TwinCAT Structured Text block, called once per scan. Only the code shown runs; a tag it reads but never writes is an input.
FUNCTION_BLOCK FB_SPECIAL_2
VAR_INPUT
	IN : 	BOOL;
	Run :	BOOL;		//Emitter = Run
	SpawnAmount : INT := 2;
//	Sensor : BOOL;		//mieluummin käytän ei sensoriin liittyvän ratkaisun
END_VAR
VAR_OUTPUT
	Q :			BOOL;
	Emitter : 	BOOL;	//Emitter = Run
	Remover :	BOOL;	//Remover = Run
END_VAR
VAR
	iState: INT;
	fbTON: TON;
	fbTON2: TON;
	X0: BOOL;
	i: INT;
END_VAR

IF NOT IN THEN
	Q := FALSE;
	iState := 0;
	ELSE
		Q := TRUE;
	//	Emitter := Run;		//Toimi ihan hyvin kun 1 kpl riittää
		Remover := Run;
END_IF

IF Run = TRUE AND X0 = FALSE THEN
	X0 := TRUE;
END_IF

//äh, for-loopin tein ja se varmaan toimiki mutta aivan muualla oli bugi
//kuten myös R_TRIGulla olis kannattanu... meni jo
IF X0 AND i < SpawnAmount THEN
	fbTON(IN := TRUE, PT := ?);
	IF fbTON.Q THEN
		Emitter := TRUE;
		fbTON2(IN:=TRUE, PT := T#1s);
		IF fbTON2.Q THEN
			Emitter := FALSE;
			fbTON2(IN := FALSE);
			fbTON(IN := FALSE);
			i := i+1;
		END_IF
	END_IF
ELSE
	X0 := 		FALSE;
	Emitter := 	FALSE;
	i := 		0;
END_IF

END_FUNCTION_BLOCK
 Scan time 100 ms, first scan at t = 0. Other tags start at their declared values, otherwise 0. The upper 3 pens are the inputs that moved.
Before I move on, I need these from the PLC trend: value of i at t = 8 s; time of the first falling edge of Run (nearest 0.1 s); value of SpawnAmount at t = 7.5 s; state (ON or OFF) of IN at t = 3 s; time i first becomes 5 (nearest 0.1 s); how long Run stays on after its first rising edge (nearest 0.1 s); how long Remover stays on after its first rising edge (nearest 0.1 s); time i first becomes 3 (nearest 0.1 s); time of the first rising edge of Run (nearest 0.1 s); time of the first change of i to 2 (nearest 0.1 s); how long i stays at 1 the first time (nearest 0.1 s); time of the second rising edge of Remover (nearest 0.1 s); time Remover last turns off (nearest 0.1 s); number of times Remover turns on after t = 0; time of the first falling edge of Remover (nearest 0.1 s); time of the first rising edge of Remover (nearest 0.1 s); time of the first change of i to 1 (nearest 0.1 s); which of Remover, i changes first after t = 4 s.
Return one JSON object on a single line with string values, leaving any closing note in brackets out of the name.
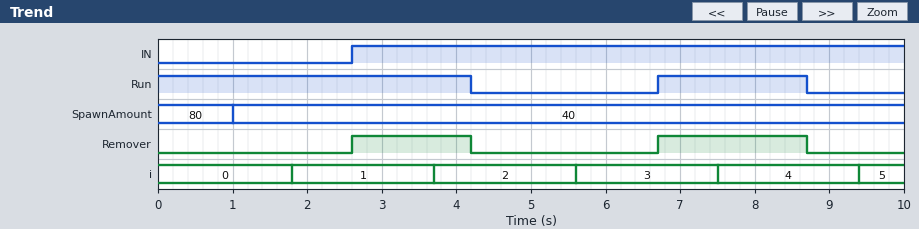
{"value of i at t = 8 s": "4", "time of the first falling edge of Run": "4.2 s", "value of SpawnAmount at t = 7.5 s": "40", "state (ON or OFF) of IN at t = 3 s": "ON", "time i first becomes 5": "9.4 s", "how long Run stays on after its first rising edge": "2.0 s", "how long Remover stays on after its first rising edge": "1.6 s", "time i first becomes 3": "5.6 s", "time of the first rising edge of Run": "6.7 s", "time of the first change of i to 2": "3.7 s", "how long i stays at 1 the first time": "1.9 s", "time of the second rising edge of Remover": "6.7 s", "time Remover last turns off": "8.7 s", "number of times Remover turns on after t = 0": "2", "time of the first falling edge of Remover": "4.2 s", "time of the first rising edge of Remover": "2.6 s", "time of the first change of i to 1": "1.8 s", "which of Remover, i changes first after t = 4 s": "Remover"}
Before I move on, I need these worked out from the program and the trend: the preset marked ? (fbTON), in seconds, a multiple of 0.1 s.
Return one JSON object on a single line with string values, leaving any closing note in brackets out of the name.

{"the preset marked ? (fbTON), in seconds, a multiple of 0.1 s": "0.8 s"}
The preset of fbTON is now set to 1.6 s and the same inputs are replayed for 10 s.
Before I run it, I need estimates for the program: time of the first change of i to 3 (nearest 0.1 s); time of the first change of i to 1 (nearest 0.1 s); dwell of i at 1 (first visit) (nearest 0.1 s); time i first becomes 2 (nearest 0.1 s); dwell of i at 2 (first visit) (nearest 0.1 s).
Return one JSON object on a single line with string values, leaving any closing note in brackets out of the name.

{"time of the first change of i to 3": "8.0 s", "time of the first change of i to 1": "2.6 s", "dwell of i at 1 (first visit)": "2.7 s", "time i first becomes 2": "5.3 s", "dwell of i at 2 (first visit)": "2.7 s"}
